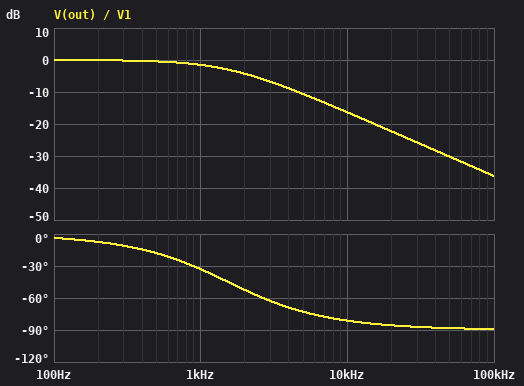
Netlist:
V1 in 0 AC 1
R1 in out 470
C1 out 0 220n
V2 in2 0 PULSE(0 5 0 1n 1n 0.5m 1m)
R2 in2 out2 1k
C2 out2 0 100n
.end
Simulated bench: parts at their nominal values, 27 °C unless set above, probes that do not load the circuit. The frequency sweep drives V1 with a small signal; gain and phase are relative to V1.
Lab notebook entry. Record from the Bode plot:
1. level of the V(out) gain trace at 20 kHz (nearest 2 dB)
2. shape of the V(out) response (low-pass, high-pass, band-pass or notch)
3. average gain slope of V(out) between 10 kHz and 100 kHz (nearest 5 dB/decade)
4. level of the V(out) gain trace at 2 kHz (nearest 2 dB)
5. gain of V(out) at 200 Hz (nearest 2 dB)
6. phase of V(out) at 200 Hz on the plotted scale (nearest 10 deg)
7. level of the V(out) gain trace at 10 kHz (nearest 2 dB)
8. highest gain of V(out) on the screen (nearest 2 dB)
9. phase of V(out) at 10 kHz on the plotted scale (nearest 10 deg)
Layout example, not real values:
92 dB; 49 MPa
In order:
-22 dB; low-pass; -20 dB/decade; -4 dB; 0 dB; -10 deg; -16 dB; 0 dB; -80 deg
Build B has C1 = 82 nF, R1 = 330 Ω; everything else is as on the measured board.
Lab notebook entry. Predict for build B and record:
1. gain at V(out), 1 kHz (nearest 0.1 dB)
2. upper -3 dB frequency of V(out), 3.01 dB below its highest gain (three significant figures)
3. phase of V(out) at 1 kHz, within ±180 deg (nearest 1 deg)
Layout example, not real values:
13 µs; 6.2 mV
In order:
-0.1 dB; 5.88 kHz; -10 deg
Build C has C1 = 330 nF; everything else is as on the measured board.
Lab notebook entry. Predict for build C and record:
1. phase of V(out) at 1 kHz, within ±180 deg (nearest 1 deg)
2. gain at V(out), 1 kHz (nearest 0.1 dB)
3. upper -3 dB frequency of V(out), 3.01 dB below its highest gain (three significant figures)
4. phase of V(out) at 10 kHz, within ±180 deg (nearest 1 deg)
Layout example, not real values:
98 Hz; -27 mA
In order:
-44 deg; -2.9 dB; 1.03 kHz; -84 deg
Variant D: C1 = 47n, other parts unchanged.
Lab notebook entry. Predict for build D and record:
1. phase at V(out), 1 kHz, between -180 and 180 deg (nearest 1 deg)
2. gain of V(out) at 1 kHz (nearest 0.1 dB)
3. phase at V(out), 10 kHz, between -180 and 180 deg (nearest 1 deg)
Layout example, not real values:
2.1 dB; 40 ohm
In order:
-8 deg; -0.1 dB; -54 deg
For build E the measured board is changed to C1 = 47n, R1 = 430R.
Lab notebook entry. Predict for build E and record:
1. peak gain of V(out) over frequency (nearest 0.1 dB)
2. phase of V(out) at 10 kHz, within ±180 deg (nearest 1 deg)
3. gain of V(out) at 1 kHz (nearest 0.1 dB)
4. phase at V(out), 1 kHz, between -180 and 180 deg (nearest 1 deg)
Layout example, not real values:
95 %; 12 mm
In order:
0 dB; -52 deg; -0.1 dB; -7 deg
